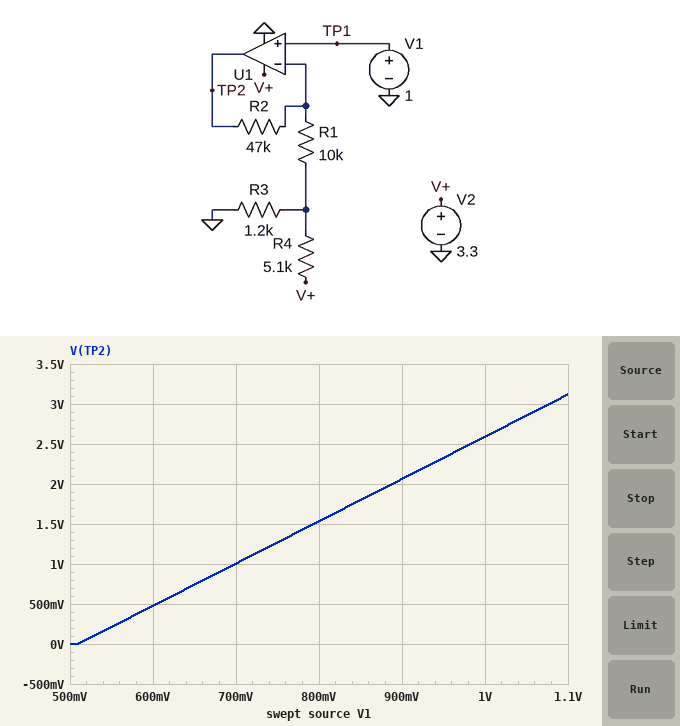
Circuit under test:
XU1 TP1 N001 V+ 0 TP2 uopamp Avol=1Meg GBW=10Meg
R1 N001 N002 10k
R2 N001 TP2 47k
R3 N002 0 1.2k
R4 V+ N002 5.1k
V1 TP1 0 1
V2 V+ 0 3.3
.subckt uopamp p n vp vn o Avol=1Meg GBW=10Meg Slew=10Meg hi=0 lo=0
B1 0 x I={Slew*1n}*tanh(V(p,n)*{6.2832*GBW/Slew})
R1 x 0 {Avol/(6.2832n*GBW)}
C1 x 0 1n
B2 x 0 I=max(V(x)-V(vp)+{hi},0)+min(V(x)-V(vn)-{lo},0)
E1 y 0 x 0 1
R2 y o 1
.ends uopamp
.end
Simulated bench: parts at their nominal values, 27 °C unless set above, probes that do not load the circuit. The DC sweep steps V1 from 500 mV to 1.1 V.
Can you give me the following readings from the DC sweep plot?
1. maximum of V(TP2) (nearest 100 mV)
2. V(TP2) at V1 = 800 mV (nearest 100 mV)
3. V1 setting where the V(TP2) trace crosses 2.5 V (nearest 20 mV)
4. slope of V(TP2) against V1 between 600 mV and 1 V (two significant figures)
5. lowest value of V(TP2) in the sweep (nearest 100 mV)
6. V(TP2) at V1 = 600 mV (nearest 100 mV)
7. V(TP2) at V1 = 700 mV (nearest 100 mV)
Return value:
3.1 V
1.5 V
980 mV
5.3 V/V
0 V
500 mV
1.0 V
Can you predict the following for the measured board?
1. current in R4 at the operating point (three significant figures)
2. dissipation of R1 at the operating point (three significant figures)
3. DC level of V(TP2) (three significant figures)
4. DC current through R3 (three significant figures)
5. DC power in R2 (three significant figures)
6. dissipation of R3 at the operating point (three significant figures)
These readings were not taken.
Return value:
517 µA
11.5 µW
2.59 V
551 µA
53.9 µW
365 µW
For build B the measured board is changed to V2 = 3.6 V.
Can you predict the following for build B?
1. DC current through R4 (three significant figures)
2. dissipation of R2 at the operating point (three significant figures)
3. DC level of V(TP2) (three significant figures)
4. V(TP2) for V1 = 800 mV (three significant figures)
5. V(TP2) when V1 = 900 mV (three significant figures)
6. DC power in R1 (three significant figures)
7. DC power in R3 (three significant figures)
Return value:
566 µA
38.6 µW
2.35 V
1.29 V
1.82 V
8.21 µW
424 µW
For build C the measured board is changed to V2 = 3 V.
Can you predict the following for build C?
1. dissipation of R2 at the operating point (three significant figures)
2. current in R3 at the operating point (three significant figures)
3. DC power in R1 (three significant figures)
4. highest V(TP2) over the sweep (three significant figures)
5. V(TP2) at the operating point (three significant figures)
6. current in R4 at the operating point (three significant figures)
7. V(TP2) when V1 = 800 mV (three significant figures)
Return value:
71.7 µW
508 µA
15.3 µW
3.00 V
2.84 V
469 µA
1.78 V
